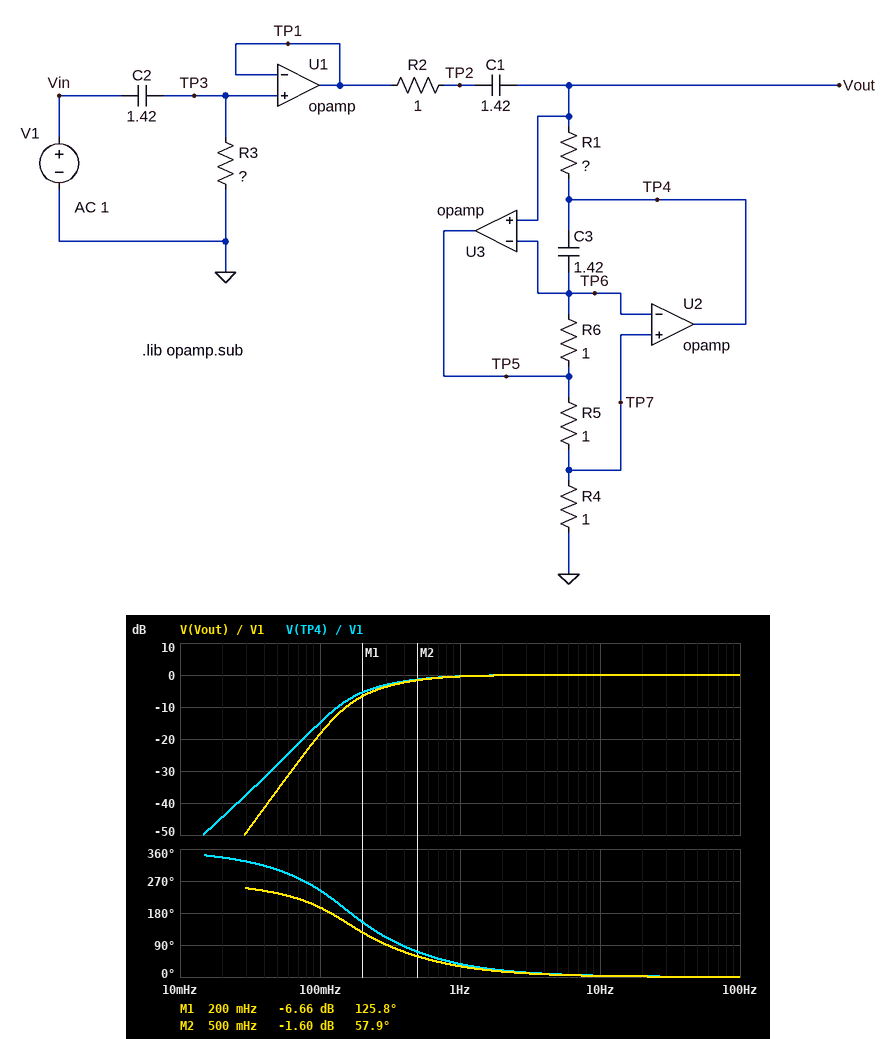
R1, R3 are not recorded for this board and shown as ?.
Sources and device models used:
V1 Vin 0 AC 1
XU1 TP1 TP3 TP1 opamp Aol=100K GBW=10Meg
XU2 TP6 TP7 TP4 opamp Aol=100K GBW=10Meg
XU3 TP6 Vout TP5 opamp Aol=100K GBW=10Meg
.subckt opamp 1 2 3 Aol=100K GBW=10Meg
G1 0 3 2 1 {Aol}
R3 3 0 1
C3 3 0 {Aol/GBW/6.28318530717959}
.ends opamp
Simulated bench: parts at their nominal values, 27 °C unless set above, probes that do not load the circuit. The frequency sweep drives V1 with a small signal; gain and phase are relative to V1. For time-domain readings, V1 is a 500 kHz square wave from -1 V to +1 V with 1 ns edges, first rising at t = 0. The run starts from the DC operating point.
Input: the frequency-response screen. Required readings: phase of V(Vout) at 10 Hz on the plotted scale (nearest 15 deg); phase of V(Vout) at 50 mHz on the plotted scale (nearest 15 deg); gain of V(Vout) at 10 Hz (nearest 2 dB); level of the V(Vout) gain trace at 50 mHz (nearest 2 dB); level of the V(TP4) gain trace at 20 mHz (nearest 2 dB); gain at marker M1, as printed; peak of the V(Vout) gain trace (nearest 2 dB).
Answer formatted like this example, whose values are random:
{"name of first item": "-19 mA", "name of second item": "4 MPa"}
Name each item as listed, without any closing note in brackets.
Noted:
{"phase of V(Vout) at 10 Hz on the plotted scale": "0 deg", "phase of V(Vout) at 50 mHz on the plotted scale": "240 deg", "gain of V(Vout) at 10 Hz": "0 dB", "level of the V(Vout) gain trace at 50 mHz": "-36 dB", "level of the V(TP4) gain trace at 20 mHz": "-44 dB", "gain at marker M1, as printed": "-6.66 dB", "peak of the V(Vout) gain trace": "0 dB"}
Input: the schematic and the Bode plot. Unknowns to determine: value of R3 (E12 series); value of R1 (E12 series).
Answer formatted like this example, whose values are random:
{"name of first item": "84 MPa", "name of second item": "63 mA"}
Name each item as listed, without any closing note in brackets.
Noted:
{"value of R3": "0.33 Ω", "value of R1": "0.56 Ω"}
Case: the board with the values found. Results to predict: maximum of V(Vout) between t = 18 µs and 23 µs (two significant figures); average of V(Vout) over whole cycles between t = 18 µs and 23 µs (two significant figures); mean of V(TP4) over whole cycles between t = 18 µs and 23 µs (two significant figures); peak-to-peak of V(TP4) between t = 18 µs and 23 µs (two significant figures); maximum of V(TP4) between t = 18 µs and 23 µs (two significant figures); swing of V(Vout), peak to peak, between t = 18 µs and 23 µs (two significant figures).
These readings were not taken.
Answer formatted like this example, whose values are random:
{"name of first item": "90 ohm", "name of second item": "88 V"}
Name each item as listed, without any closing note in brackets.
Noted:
{"maximum of V(Vout) between t = 18 µs and 23 µs": "2.0 V", "average of V(Vout) over whole cycles between t = 18 µs and 23 µs": "1.0 V", "mean of V(TP4) over whole cycles between t = 18 µs and 23 µs": "1.0 V", "peak-to-peak of V(TP4) between t = 18 µs and 23 µs": "2.0 V", "maximum of V(TP4) between t = 18 µs and 23 µs": "2.0 V", "swing of V(Vout), peak to peak, between t = 18 µs and 23 µs": "2.0 V"}
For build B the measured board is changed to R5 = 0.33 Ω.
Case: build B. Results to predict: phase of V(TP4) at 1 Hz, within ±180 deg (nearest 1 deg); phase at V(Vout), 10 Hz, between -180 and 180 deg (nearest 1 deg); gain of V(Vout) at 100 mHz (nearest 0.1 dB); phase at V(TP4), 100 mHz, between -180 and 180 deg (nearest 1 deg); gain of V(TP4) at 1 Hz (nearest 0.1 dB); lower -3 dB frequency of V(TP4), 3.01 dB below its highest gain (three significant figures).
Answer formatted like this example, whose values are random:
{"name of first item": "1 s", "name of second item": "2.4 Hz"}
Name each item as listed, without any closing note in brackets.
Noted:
{"phase of V(TP4) at 1 Hz, within ±180 deg": "25 deg", "phase at V(Vout), 10 Hz, between -180 and 180 deg": "2 deg", "gain of V(Vout) at 100 mHz": "-8.0 dB", "phase at V(TP4), 100 mHz, between -180 and 180 deg": "162 deg", "gain of V(TP4) at 1 Hz": "-0.4 dB", "lower -3 dB frequency of V(TP4), 3.01 dB below its highest gain": "300 mHz"}
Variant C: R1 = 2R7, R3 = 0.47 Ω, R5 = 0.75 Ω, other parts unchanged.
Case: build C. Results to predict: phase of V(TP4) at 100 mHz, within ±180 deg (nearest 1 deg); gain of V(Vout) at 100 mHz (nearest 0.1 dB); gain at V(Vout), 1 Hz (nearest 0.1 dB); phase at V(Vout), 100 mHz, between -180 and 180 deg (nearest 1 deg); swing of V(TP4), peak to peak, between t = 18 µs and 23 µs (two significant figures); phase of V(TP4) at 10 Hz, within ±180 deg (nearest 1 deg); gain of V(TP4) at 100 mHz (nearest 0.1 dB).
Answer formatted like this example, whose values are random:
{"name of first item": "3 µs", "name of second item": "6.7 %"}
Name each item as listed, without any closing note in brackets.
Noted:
{"phase of V(TP4) at 100 mHz, within ±180 deg": "133 deg", "gain of V(Vout) at 100 mHz": "-5.4 dB", "gain at V(Vout), 1 Hz": "-0.2 dB", "phase at V(Vout), 100 mHz, between -180 and 180 deg": "93 deg", "swing of V(TP4), peak to peak, between t = 18 µs and 23 µs": "2.1 V", "phase of V(TP4) at 10 Hz, within ±180 deg": "2 deg", "gain of V(TP4) at 100 mHz": "-3.1 dB"}
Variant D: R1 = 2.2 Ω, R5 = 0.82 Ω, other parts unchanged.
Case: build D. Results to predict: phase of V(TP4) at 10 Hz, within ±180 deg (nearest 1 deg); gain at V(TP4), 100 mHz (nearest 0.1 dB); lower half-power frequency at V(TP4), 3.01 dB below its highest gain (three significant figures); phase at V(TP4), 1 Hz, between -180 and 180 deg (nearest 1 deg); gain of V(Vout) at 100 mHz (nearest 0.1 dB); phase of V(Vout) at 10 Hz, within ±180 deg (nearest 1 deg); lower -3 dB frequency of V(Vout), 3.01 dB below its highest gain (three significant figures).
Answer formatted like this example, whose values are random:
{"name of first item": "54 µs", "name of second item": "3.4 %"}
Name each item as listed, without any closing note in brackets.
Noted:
{"phase of V(TP4) at 10 Hz, within ±180 deg": "3 deg", "gain at V(TP4), 100 mHz": "-4.9 dB", "lower half-power frequency at V(TP4), 3.01 dB below its highest gain": "284 mHz", "phase at V(TP4), 1 Hz, between -180 and 180 deg": "26 deg", "gain of V(Vout) at 100 mHz": "-7.6 dB", "phase of V(Vout) at 10 Hz, within ±180 deg": "2 deg", "lower -3 dB frequency of V(Vout), 3.01 dB below its highest gain": "315 mHz"}
